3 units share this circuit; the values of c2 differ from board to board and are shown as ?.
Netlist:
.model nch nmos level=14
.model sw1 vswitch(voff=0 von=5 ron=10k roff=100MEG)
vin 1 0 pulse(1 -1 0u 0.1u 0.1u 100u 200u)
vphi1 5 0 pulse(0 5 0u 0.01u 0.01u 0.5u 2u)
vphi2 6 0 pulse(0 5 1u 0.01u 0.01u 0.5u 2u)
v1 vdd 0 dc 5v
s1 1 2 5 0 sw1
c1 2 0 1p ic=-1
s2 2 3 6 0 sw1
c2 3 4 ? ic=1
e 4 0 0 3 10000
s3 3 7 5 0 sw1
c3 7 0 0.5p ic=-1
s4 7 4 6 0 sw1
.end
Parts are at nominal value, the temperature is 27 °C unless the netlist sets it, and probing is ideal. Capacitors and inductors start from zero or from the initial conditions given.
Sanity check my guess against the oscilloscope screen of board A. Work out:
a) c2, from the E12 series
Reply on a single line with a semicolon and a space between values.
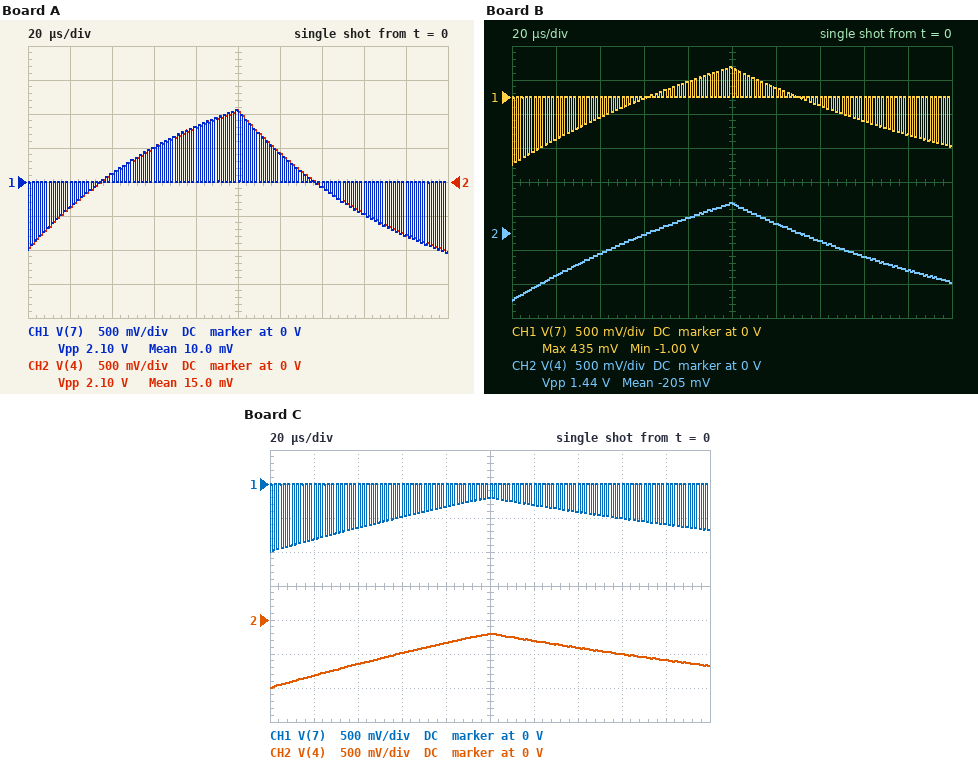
22 pF
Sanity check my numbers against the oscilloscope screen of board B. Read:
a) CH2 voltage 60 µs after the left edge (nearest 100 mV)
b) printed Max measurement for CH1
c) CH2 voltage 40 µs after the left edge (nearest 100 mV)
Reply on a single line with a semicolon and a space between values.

0 V; 435 mV; -300 mV
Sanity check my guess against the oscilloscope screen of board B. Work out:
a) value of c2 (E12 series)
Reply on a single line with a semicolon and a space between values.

39 pF
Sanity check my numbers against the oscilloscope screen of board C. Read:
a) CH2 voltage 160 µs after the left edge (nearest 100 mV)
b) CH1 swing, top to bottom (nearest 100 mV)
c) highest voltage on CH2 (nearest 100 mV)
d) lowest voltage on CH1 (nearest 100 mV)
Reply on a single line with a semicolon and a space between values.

-500 mV; 1.0 V; -200 mV; -1.0 V
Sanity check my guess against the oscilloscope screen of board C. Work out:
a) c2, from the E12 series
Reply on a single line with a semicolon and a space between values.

82 pF
